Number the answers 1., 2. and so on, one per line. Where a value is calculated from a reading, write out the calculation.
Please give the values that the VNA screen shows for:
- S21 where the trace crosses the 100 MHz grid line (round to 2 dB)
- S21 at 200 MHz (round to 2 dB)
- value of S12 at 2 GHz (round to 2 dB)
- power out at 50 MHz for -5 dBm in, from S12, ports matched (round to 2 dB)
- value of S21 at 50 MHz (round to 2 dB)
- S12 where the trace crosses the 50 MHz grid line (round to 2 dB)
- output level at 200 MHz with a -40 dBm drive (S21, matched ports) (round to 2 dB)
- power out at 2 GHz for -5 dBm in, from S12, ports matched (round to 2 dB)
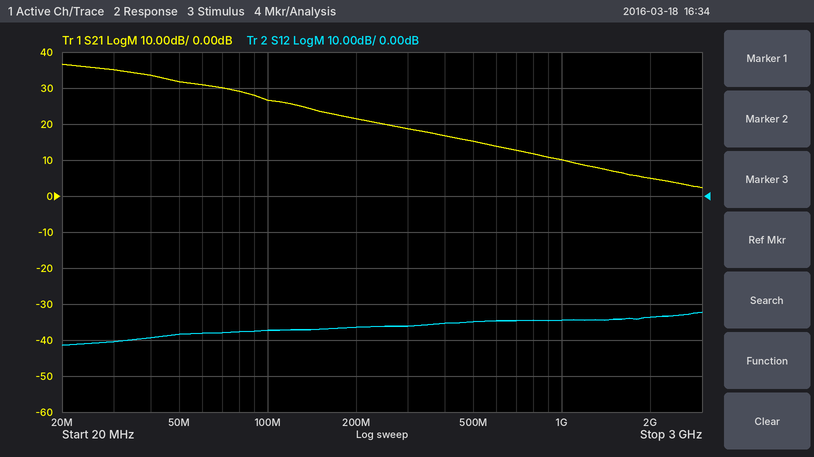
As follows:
1. 26 dB
2. 22 dB
3. -34 dB
4. -5 dBm + (-38 dB) = -44 dBm
5. 32 dB
6. -38 dB
7. -40 dBm + (22 dB) = -18 dBm
8. -5 dBm + (-34 dB) = -38 dBm
